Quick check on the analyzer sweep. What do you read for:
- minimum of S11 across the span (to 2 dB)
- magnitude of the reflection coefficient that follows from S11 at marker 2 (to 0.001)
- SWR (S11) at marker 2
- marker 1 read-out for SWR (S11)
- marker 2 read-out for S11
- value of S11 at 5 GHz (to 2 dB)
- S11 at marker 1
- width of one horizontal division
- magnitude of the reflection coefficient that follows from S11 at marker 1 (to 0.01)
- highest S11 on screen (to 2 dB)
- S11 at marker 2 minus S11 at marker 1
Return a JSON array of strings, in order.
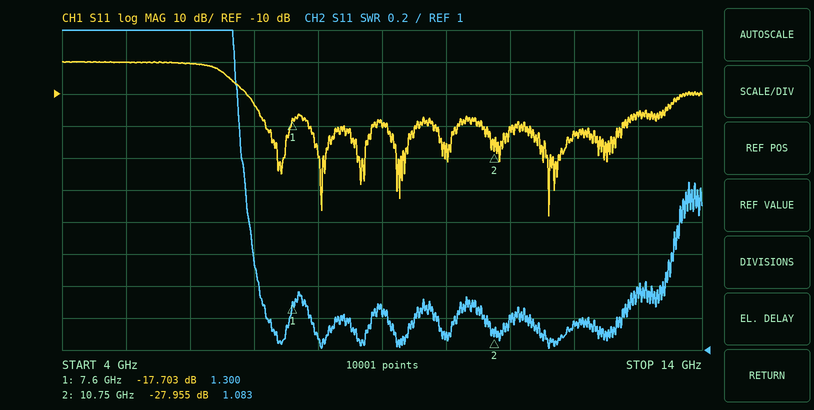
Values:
["-48 dB", "0.040", "1.083", "1.300", "-27.955 dB", "0 dB", "-17.703 dB", "1 GHz", "0.13", "0 dB", "-10.252 dB"]
